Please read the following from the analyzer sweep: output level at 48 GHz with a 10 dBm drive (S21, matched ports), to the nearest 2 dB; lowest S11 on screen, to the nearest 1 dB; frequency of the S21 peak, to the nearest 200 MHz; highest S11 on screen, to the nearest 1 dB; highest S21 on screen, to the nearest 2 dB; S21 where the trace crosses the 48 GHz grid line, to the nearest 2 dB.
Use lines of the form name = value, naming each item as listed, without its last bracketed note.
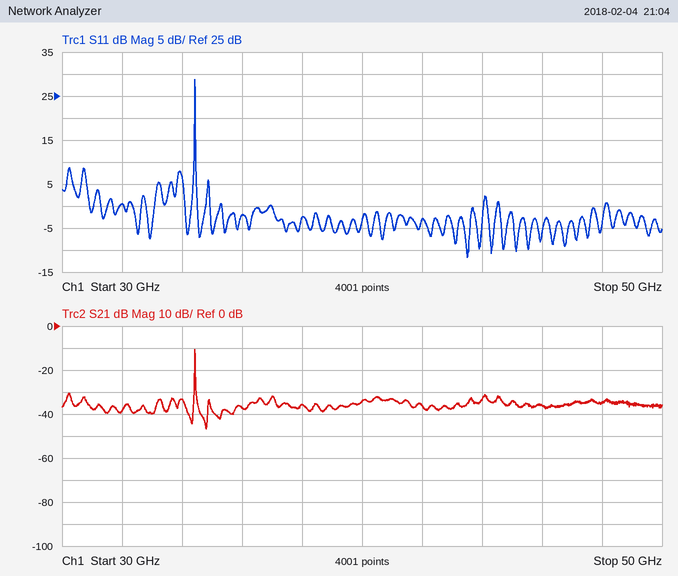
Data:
output level at 48 GHz with a 10 dBm drive (S21, matched ports), to the nearest 2 dB = -24 dBm
lowest S11 on screen, to the nearest 1 dB = -12 dB
frequency of the S21 peak, to the nearest 200 MHz = 34.4 GHz
highest S11 on screen, to the nearest 1 dB = 29 dB
highest S21 on screen, to the nearest 2 dB = -10 dB
S21 where the trace crosses the 48 GHz grid line, to the nearest 2 dB = -34 dB
